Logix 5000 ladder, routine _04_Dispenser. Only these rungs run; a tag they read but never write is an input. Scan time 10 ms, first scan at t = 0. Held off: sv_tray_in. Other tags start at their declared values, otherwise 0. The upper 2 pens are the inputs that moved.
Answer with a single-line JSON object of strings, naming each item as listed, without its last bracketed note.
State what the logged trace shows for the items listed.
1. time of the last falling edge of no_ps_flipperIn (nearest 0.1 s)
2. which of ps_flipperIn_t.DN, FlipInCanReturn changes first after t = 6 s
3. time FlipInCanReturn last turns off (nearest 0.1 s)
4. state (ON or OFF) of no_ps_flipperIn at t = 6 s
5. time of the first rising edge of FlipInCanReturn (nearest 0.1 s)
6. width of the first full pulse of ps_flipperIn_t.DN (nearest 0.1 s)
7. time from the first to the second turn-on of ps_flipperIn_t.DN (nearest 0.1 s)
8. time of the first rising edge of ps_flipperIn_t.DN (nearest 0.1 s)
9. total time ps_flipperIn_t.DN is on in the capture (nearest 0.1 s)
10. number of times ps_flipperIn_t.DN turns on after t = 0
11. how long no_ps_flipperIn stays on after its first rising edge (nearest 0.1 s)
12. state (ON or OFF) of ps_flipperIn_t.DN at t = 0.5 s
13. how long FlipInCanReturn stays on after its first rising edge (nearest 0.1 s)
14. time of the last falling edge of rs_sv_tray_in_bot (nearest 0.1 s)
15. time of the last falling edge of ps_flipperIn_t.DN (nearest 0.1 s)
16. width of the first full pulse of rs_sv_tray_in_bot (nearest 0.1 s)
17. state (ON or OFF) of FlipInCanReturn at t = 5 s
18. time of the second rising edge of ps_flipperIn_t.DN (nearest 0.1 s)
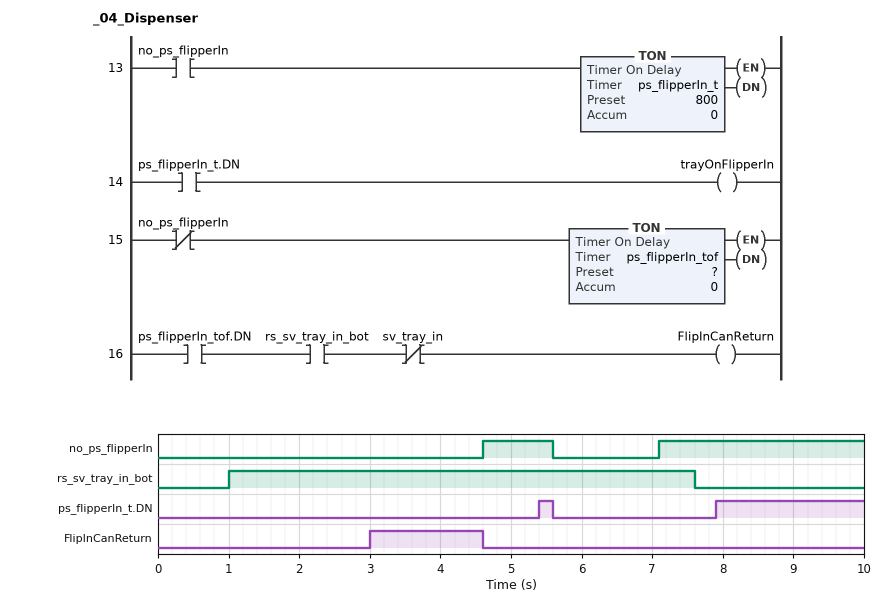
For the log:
{"time of the last falling edge of no_ps_flipperIn": "5.6 s", "which of ps_flipperIn_t.DN, FlipInCanReturn changes first after t = 6 s": "ps_flipperIn_t.DN", "time FlipInCanReturn last turns off": "4.6 s", "state (ON or OFF) of no_ps_flipperIn at t = 6 s": "OFF", "time of the first rising edge of FlipInCanReturn": "3.0 s", "width of the first full pulse of ps_flipperIn_t.DN": "0.2 s", "time from the first to the second turn-on of ps_flipperIn_t.DN": "2.5 s", "time of the first rising edge of ps_flipperIn_t.DN": "5.4 s", "total time ps_flipperIn_t.DN is on in the capture": "2.3 s", "number of times ps_flipperIn_t.DN turns on after t = 0": "2", "how long no_ps_flipperIn stays on after its first rising edge": "1.0 s", "state (ON or OFF) of ps_flipperIn_t.DN at t = 0.5 s": "OFF", "how long FlipInCanReturn stays on after its first rising edge": "1.6 s", "time of the last falling edge of rs_sv_tray_in_bot": "7.6 s", "time of the last falling edge of ps_flipperIn_t.DN": "5.6 s", "width of the first full pulse of rs_sv_tray_in_bot": "6.6 s", "state (ON or OFF) of FlipInCanReturn at t = 5 s": "OFF", "time of the second rising edge of ps_flipperIn_t.DN": "7.9 s"}
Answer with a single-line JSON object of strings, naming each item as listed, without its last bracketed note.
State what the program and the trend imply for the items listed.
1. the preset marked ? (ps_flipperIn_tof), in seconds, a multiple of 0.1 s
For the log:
{"the preset marked ? (ps_flipperIn_tof), in seconds, a multiple of 0.1 s": "3.0 s"}
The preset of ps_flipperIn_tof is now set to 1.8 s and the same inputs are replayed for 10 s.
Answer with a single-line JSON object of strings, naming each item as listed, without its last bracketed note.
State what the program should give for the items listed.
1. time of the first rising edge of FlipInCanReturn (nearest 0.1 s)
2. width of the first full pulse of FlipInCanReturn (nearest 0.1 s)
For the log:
{"time of the first rising edge of FlipInCanReturn": "1.8 s", "width of the first full pulse of FlipInCanReturn": "2.8 s"}
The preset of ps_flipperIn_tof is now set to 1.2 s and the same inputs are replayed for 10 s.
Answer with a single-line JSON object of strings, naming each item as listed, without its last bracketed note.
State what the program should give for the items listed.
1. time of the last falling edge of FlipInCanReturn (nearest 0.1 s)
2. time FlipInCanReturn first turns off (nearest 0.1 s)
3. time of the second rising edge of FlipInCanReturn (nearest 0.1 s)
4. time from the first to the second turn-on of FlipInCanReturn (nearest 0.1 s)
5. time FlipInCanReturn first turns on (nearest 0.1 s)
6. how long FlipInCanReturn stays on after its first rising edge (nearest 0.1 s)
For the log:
{"time of the last falling edge of FlipInCanReturn": "7.1 s", "time FlipInCanReturn first turns off": "4.6 s", "time of the second rising edge of FlipInCanReturn": "6.8 s", "time from the first to the second turn-on of FlipInCanReturn": "5.6 s", "time FlipInCanReturn first turns on": "1.2 s", "how long FlipInCanReturn stays on after its first rising edge": "3.4 s"}
